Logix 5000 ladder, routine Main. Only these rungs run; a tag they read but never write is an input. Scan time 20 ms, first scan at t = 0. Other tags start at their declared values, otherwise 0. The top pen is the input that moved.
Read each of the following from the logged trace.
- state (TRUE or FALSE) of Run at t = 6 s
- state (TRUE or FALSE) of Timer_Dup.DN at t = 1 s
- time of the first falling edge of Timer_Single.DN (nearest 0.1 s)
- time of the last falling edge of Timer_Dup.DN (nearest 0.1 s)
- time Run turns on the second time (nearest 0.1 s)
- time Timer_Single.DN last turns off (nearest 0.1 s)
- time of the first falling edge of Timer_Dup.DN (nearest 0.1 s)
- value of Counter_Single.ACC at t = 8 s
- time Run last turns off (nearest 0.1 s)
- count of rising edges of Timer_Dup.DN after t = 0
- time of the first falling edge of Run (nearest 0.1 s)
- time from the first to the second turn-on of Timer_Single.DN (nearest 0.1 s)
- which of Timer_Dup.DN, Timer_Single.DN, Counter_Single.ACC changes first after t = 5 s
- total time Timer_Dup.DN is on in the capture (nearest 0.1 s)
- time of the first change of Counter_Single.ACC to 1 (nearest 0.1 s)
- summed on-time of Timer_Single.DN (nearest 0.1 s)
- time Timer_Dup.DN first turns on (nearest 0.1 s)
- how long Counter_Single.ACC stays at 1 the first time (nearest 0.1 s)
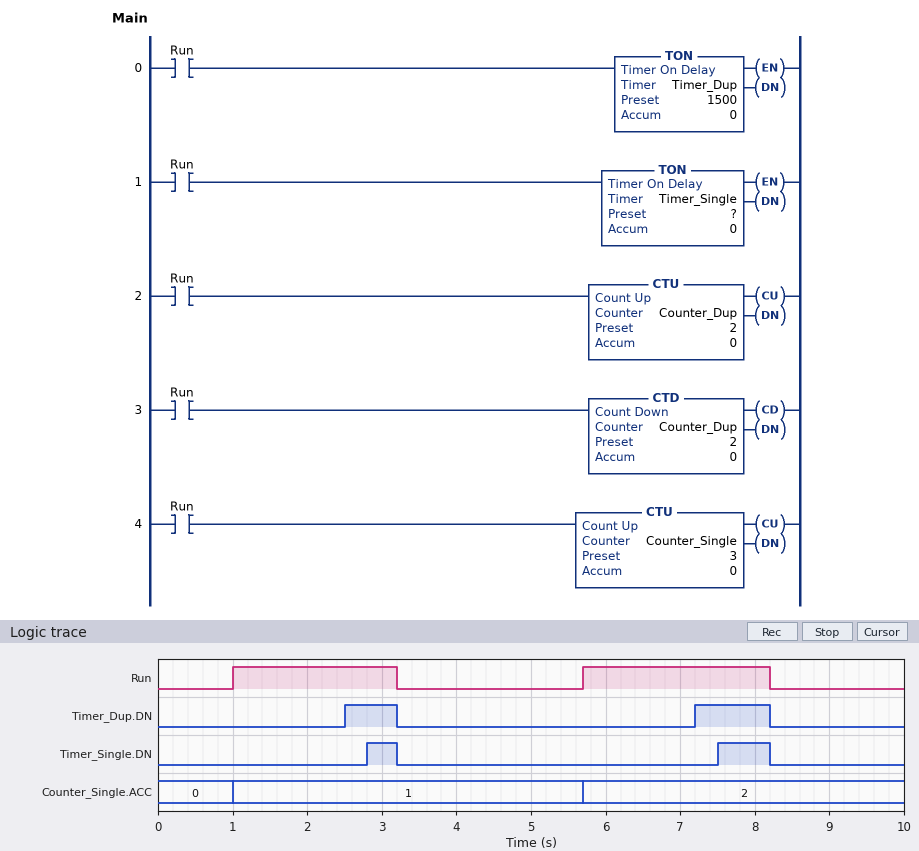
TRUE
FALSE
3.2 s
8.2 s
5.7 s
8.2 s
3.2 s
2
8.2 s
2
3.2 s
4.7 s
Counter_Single.ACC
1.7 s
1.0 s
1.1 s
2.5 s
4.7 s
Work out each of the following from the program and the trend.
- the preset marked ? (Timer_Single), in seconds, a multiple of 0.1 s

1.8 s
